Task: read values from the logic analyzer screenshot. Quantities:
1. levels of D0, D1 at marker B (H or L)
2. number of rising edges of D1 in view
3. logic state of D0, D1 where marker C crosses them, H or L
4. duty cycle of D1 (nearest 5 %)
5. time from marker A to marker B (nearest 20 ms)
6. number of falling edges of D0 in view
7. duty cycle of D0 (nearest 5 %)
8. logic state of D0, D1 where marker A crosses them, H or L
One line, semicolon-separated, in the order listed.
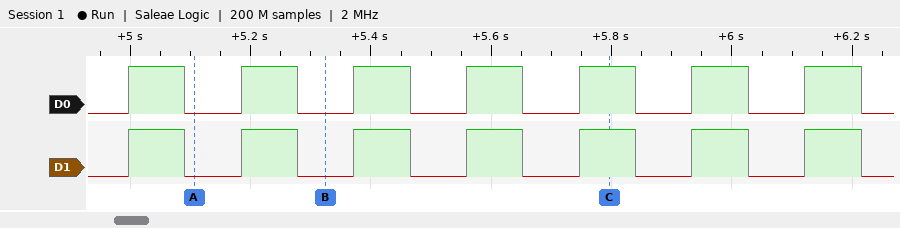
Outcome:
D0=L, D1=L; 7; D0=H, D1=H; 50 %; 220 ms; 7; 50 %; D0=L, D1=L
